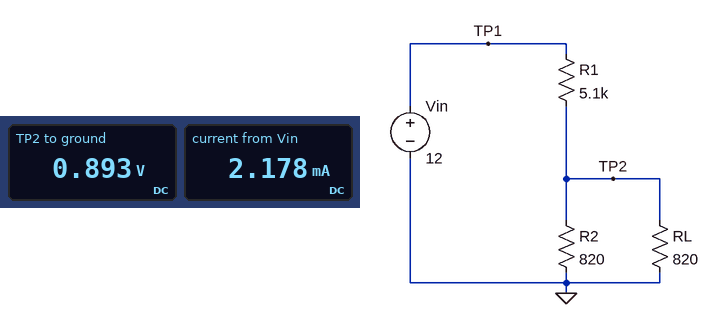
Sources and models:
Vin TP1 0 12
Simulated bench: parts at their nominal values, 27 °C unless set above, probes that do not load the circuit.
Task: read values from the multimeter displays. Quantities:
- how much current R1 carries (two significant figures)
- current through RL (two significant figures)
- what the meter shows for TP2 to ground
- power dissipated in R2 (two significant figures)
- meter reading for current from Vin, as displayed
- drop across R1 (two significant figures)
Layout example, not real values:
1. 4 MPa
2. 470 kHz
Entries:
1. 2.2 mA
2. 1.1 mA
3. 0.893 V
4. 970 µW
5. 2.178 mA
6. 11 V
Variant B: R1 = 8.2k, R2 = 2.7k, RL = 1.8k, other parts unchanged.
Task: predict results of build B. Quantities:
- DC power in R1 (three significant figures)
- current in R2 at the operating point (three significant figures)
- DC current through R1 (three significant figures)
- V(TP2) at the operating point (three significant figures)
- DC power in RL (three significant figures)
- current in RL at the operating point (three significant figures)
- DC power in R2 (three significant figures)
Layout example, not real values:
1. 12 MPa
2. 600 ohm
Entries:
1. 13.7 mW
2. 517 µA
3. 1.29 mA
4. 1.40 V
5. 1.08 mW
6. 776 µA
7. 722 µW
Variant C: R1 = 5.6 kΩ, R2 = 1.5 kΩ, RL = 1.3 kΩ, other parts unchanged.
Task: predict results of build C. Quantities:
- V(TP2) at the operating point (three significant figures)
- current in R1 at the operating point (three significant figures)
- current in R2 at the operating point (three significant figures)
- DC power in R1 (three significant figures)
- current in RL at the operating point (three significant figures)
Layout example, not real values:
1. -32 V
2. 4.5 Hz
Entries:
1. 1.33 V
2. 1.91 mA
3. 885 µA
4. 20.3 mW
5. 1.02 mA
